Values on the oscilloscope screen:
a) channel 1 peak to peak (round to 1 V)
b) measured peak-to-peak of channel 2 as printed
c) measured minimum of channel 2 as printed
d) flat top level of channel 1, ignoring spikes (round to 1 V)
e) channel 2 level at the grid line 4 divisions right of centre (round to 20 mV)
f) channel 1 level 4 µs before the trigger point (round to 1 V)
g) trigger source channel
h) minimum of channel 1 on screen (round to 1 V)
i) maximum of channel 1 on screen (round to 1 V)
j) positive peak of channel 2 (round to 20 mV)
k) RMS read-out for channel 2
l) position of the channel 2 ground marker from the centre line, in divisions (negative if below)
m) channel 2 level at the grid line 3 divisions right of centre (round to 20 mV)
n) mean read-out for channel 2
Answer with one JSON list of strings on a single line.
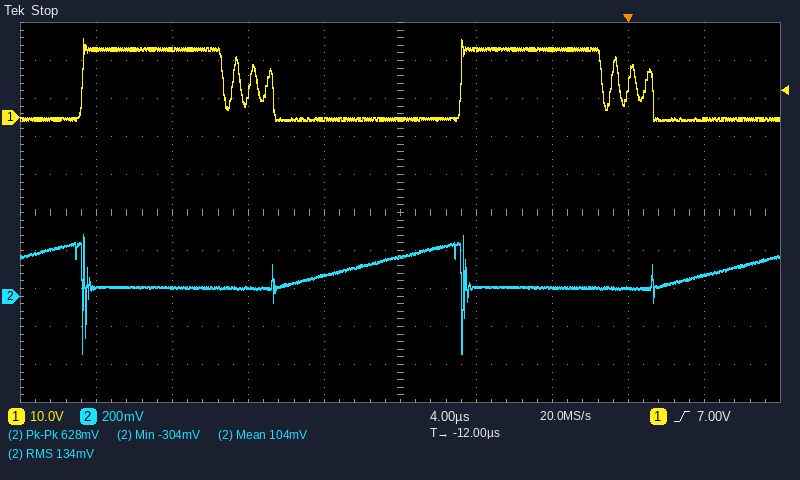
["22 V", "628 mV", "-304 mV", "18 V", "120 mV", "18 V", "channel 1", "-1 V", "21 V", "320 mV", "134 mV", "-2.2 div", "40 mV", "104 mV"]
